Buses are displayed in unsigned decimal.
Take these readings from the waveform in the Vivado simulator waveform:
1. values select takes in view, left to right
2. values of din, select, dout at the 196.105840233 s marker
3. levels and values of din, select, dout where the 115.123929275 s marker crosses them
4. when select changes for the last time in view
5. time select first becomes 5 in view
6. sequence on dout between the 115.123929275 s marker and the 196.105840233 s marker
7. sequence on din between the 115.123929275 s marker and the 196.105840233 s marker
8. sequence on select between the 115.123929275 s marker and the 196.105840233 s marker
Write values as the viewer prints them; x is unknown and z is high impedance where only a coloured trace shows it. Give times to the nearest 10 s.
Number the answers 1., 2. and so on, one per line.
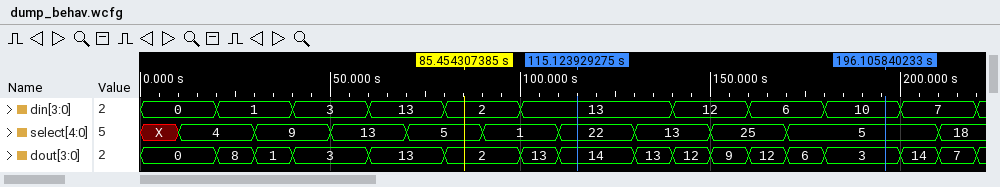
1. X, 4, 9, 13, 5, 1, 22, 13, 25, 5, 18
2. din=10, select=5, dout=3
3. din=13, select=22, dout=14
4. 210 s
5. 70 s
6. 14, 13, 12, 9, 12, 6, 3
7. 13, 12, 6, 10
8. 22, 13, 25, 5
